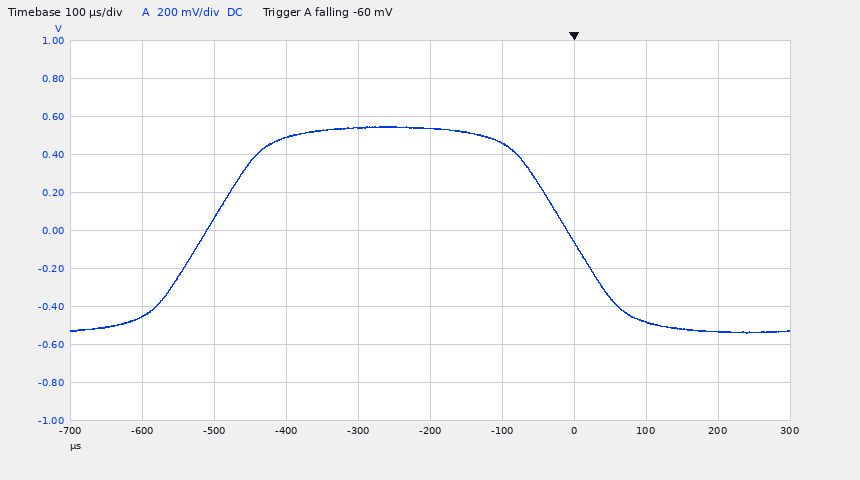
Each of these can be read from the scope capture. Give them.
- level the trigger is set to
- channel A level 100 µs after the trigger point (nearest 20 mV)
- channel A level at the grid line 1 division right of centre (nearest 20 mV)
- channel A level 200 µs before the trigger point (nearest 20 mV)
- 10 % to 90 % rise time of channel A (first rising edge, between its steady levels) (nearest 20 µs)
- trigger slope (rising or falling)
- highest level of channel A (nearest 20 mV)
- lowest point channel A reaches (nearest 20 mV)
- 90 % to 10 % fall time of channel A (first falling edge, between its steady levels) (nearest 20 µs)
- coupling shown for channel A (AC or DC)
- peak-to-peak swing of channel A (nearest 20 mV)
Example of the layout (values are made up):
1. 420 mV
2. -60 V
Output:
1. -60 mV
2. -480 mV
3. 460 mV
4. 540 mV
5. 160 µs
6. falling
7. 540 mV
8. -540 mV
9. 160 µs
10. DC
11. 1.08 V
